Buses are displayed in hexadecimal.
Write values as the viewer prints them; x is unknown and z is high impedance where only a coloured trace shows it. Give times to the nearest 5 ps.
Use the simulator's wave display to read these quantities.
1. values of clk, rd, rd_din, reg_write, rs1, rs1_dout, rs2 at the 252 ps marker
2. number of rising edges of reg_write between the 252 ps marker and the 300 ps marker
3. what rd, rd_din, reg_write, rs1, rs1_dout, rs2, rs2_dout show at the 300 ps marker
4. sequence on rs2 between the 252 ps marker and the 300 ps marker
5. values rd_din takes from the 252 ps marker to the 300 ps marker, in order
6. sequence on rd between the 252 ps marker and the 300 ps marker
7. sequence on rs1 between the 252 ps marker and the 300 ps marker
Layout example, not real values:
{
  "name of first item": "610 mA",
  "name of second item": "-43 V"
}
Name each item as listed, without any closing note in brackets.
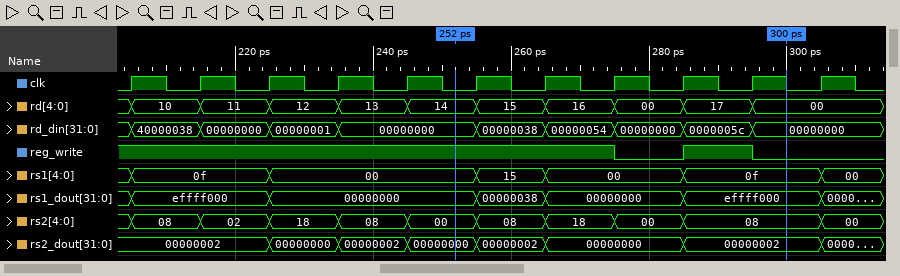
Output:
{
  "values of clk, rd, rd_din, reg_write, rs1, rs1_dout, rs2 at the 252 ps marker": "clk=0, rd=14, rd_din=00000000, reg_write=1, rs1=00, rs1_dout=00000000, rs2=00",
  "number of rising edges of reg_write between the 252 ps marker and the 300 ps marker": "1",
  "what rd, rd_din, reg_write, rs1, rs1_dout, rs2, rs2_dout show at the 300 ps marker": "rd=00, rd_din=00000000, reg_write=0, rs1=0f, rs1_dout=effff000, rs2=08, rs2_dout=00000002",
  "sequence on rs2 between the 252 ps marker and the 300 ps marker": "00, 08, 18, 00, 08",
  "values rd_din takes from the 252 ps marker to the 300 ps marker, in order": "00000000, 00000038, 00000054, 00000000, 0000005c, 00000000",
  "sequence on rd between the 252 ps marker and the 300 ps marker": "14, 15, 16, 00, 17, 00",
  "sequence on rs1 between the 252 ps marker and the 300 ps marker": "00, 15, 00, 0f"
}
